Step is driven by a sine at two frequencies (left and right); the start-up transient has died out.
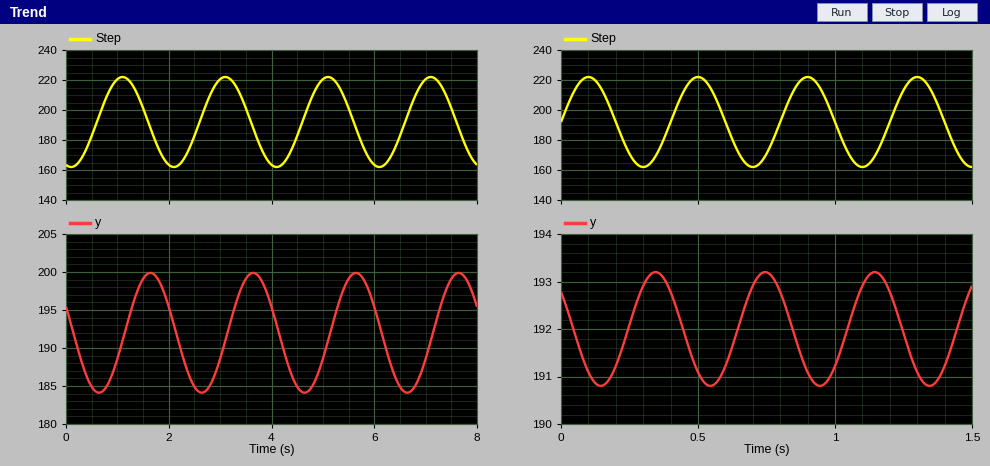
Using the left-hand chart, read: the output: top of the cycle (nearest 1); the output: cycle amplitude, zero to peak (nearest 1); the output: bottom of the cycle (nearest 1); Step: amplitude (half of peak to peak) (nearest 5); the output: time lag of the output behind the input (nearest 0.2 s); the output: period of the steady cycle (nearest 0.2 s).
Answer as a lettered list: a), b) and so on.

a) 200
b) 8
c) 184
d) 30
e) 0.6 s
f) 2.0 s
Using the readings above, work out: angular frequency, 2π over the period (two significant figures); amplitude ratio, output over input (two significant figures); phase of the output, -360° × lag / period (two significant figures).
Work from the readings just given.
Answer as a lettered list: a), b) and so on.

a) 3.1 rad/s
b) 0.27
c) -110°
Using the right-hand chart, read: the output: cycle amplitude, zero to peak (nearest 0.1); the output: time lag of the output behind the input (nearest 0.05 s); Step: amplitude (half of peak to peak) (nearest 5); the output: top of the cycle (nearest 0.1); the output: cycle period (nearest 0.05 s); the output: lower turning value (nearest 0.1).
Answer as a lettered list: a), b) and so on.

a) 1.2
b) 0.25 s
c) 30
d) 193.2
e) 0.40 s
f) 190.8
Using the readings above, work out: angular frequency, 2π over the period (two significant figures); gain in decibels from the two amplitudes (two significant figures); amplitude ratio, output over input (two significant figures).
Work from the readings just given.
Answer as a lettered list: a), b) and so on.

a) 16 rad/s
b) -28 dB
c) 0.040
